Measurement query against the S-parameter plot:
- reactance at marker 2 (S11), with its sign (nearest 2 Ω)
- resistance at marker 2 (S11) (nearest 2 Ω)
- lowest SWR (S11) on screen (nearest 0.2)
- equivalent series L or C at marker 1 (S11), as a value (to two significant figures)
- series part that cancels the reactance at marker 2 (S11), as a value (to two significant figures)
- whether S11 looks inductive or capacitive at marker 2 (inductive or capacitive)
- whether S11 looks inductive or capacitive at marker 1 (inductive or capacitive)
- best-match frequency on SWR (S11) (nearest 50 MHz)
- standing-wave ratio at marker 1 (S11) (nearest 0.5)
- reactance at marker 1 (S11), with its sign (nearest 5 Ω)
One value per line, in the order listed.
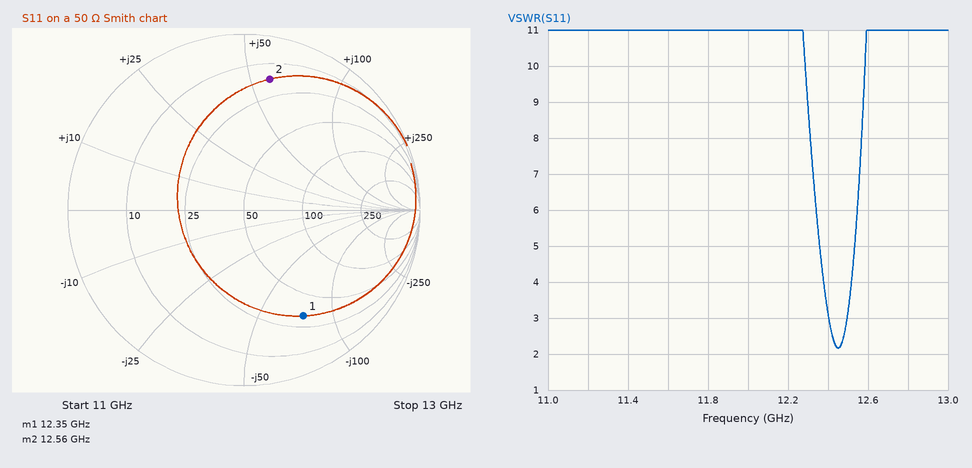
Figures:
+58 Ω
16 Ω
2.2
170 fF
220 fF
inductive
capacitive
12.45 GHz
5.5
-75 Ω
